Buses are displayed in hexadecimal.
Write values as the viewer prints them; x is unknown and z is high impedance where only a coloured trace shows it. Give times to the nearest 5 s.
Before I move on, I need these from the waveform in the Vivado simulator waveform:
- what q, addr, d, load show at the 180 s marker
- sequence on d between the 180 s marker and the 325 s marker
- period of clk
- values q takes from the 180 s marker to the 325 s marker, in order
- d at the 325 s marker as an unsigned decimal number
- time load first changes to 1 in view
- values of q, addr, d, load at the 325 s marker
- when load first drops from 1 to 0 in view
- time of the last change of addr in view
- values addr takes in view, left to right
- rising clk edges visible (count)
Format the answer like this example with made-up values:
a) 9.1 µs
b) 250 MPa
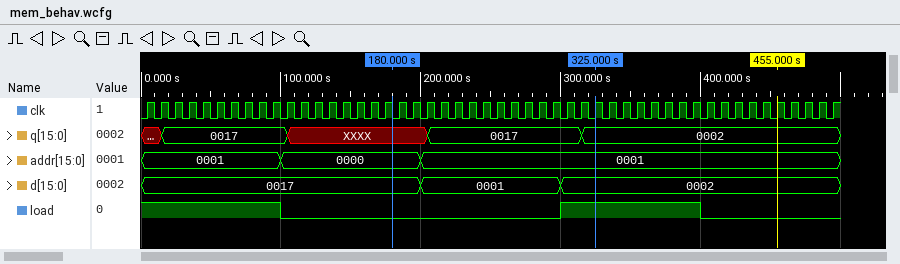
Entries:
a) q=XXXX, addr=0000, d=0017, load=0
b) 0017, 0001, 0002
c) 10 s
d) XXXX, 0017, 0002
e) 2
f) 300 s
g) q=0002, addr=0001, d=0002, load=1
h) 100 s
i) 200 s
j) 0001, 0000, 0001
k) 50
